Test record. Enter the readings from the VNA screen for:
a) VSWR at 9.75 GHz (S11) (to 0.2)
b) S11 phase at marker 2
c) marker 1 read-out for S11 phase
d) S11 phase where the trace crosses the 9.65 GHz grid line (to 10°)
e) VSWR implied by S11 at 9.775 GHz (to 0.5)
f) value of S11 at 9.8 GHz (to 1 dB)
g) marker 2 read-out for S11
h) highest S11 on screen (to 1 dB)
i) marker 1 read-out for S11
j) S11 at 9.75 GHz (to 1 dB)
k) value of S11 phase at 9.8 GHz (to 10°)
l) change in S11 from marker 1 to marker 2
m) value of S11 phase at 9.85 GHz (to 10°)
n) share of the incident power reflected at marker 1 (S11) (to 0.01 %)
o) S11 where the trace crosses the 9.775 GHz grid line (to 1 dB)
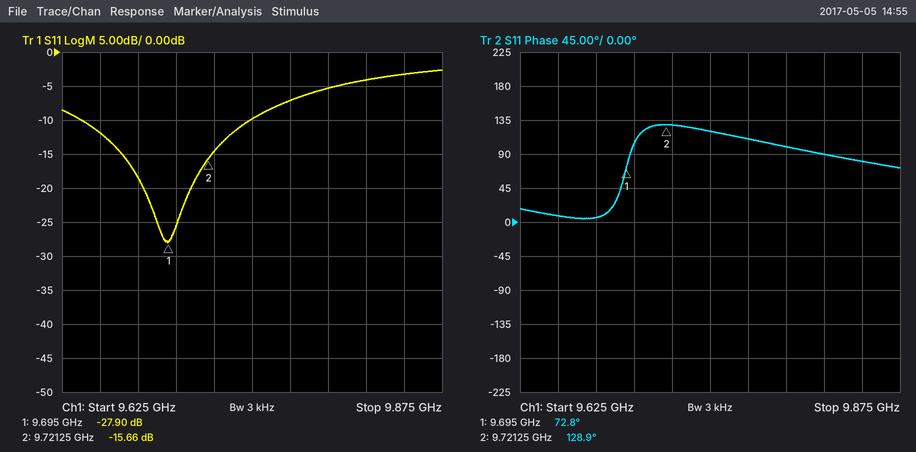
2.0
128.9°
72.8°
10°
2.5
-5 dB
-15.66 dB
-3 dB
-27.90 dB
-10 dB
100°
12.24 dB
80°
0.16 %
-7 dB
